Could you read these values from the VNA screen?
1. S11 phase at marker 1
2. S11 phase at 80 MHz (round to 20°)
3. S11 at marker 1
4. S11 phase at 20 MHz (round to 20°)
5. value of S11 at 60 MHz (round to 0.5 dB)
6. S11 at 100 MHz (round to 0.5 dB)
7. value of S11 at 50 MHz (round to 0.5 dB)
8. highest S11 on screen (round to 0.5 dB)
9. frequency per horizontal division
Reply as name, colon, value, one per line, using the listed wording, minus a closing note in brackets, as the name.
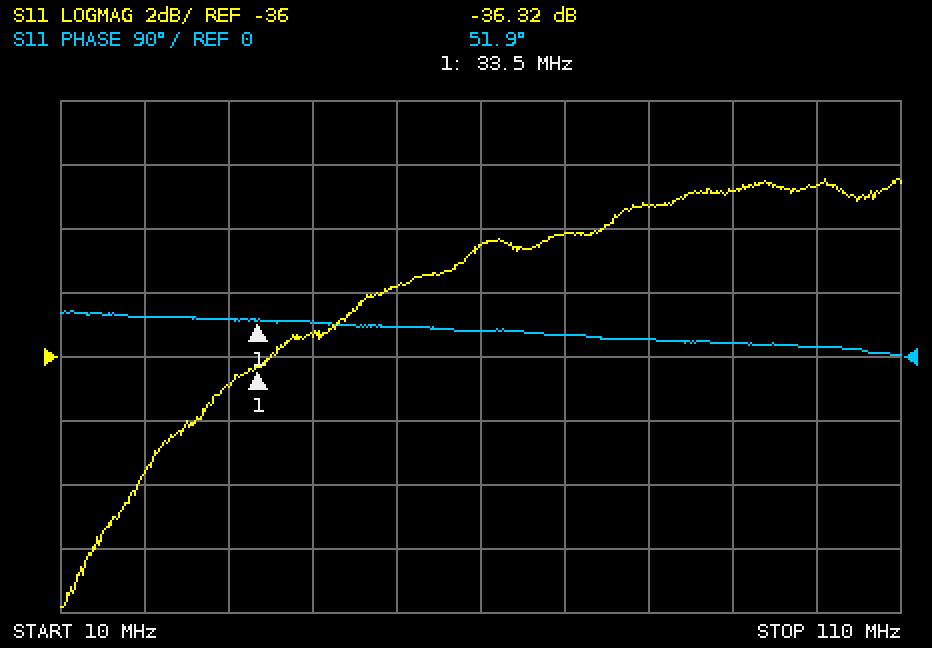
S11 phase at marker 1: 51.9°
S11 phase at 80 MHz: 20°
S11 at marker 1: -36.32 dB
S11 phase at 20 MHz: 60°
value of S11 at 60 MHz: -32.5 dB
S11 at 100 MHz: -30.5 dB
value of S11 at 50 MHz: -34.0 dB
highest S11 on screen: -30.5 dB
frequency per horizontal division: 10 MHz
